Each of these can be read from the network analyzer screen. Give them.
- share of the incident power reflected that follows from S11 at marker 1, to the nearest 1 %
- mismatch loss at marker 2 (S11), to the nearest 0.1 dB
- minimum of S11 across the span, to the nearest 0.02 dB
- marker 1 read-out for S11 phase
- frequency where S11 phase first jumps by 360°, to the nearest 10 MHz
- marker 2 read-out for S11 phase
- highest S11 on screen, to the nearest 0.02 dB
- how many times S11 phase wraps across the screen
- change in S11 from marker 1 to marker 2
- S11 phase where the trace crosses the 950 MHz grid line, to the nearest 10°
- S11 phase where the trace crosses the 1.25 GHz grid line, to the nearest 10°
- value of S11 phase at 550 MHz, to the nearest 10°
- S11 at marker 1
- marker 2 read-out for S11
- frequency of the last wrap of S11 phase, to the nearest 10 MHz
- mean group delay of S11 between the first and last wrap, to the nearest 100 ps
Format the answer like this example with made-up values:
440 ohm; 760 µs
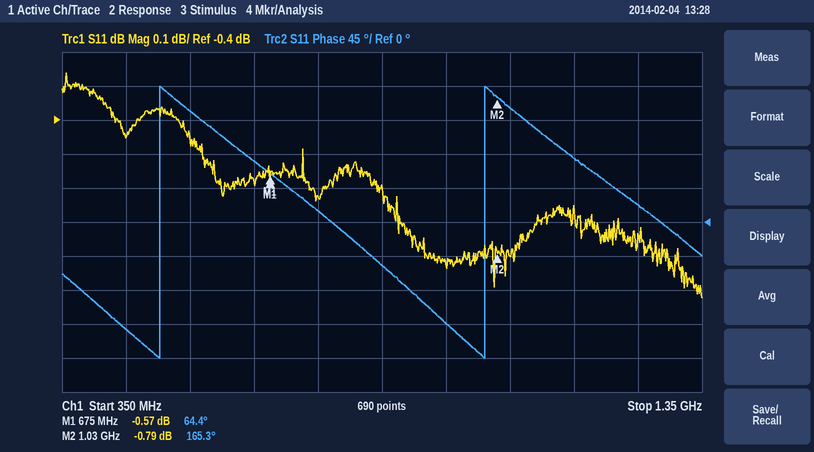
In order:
88 %; 7.8 dB; -0.92 dB; 64.4°; 500 MHz; 165.3°; -0.26 dB; 2; -0.22 dB; -130°; 20°; 150°; -0.57 dB; -0.79 dB; 1.01 GHz; 2.0 ns
